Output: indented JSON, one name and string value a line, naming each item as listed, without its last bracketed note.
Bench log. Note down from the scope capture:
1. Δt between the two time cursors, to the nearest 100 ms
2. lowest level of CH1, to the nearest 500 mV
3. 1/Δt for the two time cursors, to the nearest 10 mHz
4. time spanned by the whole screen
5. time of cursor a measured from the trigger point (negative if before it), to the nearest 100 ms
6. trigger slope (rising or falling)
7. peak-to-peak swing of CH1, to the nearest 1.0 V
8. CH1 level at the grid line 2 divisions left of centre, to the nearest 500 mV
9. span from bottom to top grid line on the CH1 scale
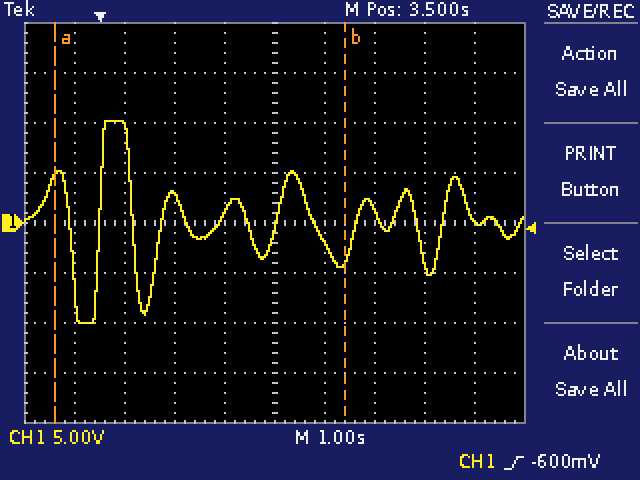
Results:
{
  "Δt between the two time cursors, to the nearest 100 ms": "5.8 s",
  "lowest level of CH1, to the nearest 500 mV": "-10.0 V",
  "1/Δt for the two time cursors, to the nearest 10 mHz": "170 mHz",
  "time spanned by the whole screen": "10 s",
  "time of cursor a measured from the trigger point (negative if before it), to the nearest 100 ms": "-900 ms",
  "trigger slope": "rising",
  "peak-to-peak swing of CH1, to the nearest 1.0 V": "20.0 V",
  "CH1 level at the grid line 2 divisions left of centre, to the nearest 500 mV": "2.5 V",
  "span from bottom to top grid line on the CH1 scale": "40 V"
}
